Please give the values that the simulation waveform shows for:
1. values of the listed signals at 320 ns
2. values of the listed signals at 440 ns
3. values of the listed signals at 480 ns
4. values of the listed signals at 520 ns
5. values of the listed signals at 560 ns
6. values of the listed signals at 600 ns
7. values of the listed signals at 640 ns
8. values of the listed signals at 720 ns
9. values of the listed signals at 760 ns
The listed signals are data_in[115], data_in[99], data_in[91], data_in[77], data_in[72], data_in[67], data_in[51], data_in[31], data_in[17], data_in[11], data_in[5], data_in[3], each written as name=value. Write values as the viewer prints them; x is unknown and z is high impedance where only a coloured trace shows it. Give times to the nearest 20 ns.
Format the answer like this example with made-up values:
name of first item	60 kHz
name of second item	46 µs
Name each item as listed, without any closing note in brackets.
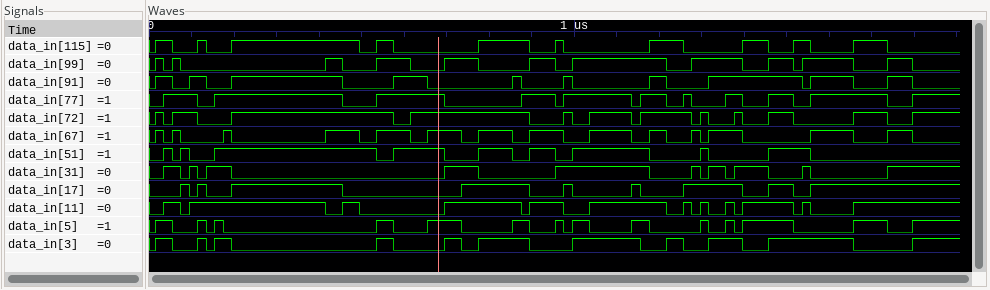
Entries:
values of the listed signals at 320 ns	data_in[115]=1, data_in[99]=0, data_in[91]=1, data_in[77]=1, data_in[72]=1, data_in[67]=0, data_in[51]=1, data_in[31]=0, data_in[17]=1, data_in[11]=1, data_in[5]=0, data_in[3]=0
values of the listed signals at 440 ns	data_in[115]=1, data_in[99]=1, data_in[91]=1, data_in[77]=1, data_in[72]=1, data_in[67]=1, data_in[51]=1, data_in[31]=0, data_in[17]=1, data_in[11]=0, data_in[5]=0, data_in[3]=0
values of the listed signals at 480 ns	data_in[115]=1, data_in[99]=0, data_in[91]=0, data_in[77]=0, data_in[72]=1, data_in[67]=1, data_in[51]=1, data_in[31]=0, data_in[17]=0, data_in[11]=1, data_in[5]=0, data_in[3]=0
values of the listed signals at 520 ns	data_in[115]=0, data_in[99]=0, data_in[91]=0, data_in[77]=0, data_in[72]=1, data_in[67]=0, data_in[51]=1, data_in[31]=0, data_in[17]=0, data_in[11]=0, data_in[5]=0, data_in[3]=0
values of the listed signals at 560 ns	data_in[115]=1, data_in[99]=1, data_in[91]=0, data_in[77]=1, data_in[72]=1, data_in[67]=1, data_in[51]=0, data_in[31]=0, data_in[17]=0, data_in[11]=0, data_in[5]=1, data_in[3]=1
values of the listed signals at 600 ns	data_in[115]=0, data_in[99]=1, data_in[91]=1, data_in[77]=1, data_in[72]=0, data_in[67]=1, data_in[51]=1, data_in[31]=0, data_in[17]=0, data_in[11]=0, data_in[5]=0, data_in[3]=0
values of the listed signals at 640 ns	data_in[115]=0, data_in[99]=0, data_in[91]=1, data_in[77]=1, data_in[72]=1, data_in[67]=0, data_in[51]=1, data_in[31]=0, data_in[17]=0, data_in[11]=0, data_in[5]=0, data_in[3]=0
values of the listed signals at 720 ns	data_in[115]=0, data_in[99]=1, data_in[91]=0, data_in[77]=0, data_in[72]=1, data_in[67]=1, data_in[51]=0, data_in[31]=1, data_in[17]=0, data_in[11]=1, data_in[5]=1, data_in[3]=1
values of the listed signals at 760 ns	data_in[115]=0, data_in[99]=1, data_in[91]=0, data_in[77]=0, data_in[72]=1, data_in[67]=0, data_in[51]=0, data_in[31]=1, data_in[17]=1, data_in[11]=1, data_in[5]=0, data_in[3]=0
